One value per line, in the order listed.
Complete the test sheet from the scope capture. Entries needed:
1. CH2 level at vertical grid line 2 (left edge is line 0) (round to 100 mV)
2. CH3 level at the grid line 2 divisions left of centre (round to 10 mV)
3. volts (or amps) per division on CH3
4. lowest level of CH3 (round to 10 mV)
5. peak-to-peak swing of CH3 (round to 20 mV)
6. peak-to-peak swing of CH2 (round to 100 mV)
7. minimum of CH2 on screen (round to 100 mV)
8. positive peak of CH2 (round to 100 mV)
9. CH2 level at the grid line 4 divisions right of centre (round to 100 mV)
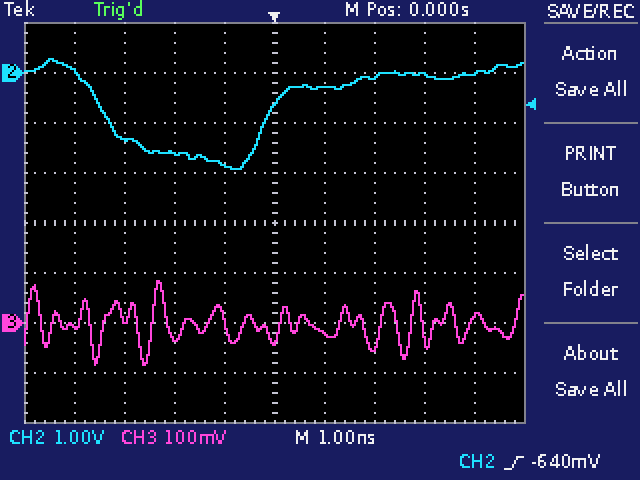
-1.3 V
-30 mV
100 mV
-80 mV
160 mV
2.2 V
-1.9 V
300 mV
0.0 V
